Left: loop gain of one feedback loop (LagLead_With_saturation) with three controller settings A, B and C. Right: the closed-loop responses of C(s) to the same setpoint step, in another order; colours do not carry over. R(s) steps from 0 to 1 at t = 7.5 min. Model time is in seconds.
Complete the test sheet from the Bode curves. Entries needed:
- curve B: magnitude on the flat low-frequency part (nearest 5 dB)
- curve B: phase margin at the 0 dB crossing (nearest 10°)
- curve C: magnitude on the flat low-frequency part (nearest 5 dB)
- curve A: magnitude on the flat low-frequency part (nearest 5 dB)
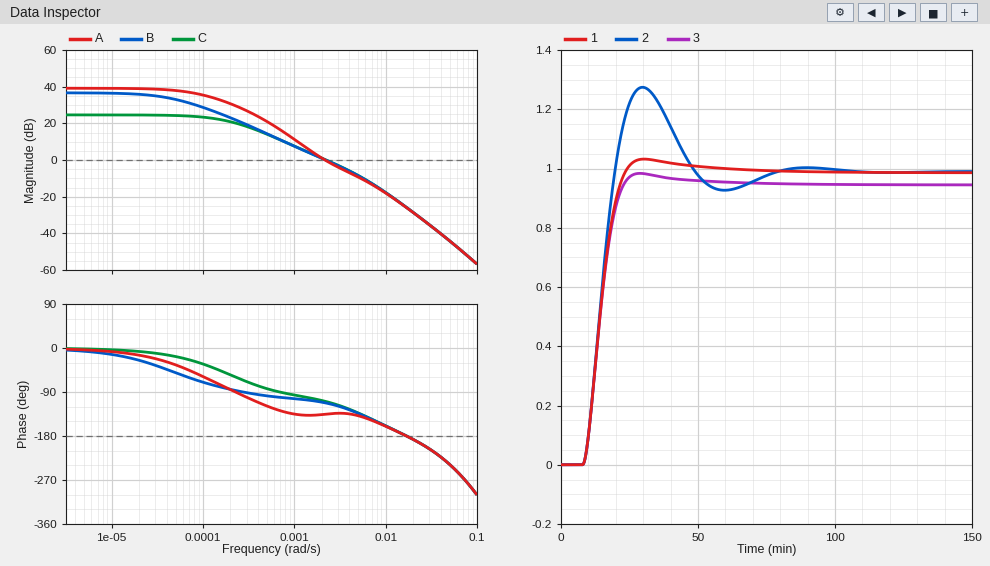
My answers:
35 dB
70°
25 dB
40 dB
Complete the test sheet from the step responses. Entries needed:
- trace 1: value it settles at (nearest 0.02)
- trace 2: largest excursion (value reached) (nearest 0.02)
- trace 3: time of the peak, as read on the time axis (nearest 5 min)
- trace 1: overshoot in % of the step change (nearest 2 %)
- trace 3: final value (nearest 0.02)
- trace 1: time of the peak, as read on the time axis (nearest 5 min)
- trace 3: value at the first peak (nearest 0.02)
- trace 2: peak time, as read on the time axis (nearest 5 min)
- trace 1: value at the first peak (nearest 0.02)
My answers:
0.98
1.28
30 min
4 %
0.94
30 min
0.98
30 min
1.04
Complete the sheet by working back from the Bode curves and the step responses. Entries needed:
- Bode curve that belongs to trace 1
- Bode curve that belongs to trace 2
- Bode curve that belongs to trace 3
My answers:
B
A
C
